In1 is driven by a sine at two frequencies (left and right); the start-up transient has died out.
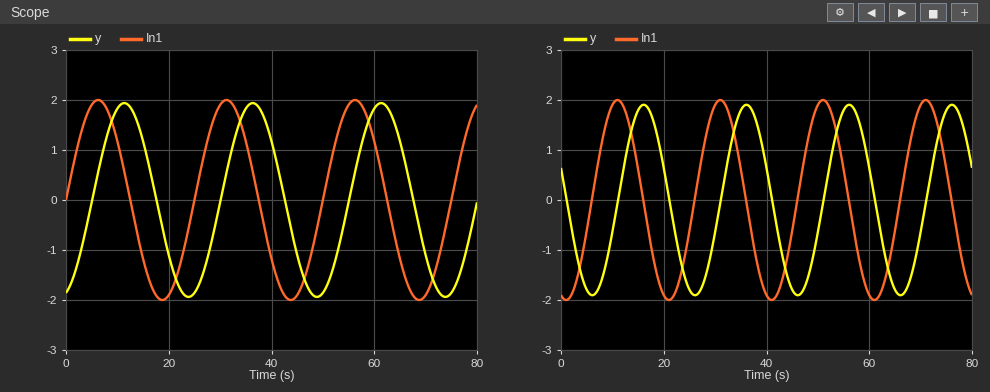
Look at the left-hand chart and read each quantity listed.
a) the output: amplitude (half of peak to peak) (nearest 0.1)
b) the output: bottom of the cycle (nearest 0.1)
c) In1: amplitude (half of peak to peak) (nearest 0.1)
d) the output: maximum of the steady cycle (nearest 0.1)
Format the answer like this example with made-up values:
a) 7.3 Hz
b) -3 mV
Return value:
a) 1.9
b) -1.9
c) 2.0
d) 1.9
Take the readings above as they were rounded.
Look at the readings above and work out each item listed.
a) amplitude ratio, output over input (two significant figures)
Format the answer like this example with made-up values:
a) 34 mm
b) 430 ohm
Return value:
a) 0.95
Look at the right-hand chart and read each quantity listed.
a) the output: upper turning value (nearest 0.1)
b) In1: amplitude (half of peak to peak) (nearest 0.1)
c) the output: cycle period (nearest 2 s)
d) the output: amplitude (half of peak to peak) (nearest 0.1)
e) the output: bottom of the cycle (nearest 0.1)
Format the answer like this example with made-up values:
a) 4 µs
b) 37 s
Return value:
a) 1.9
b) 2.0
c) 20 s
d) 1.9
e) -1.9
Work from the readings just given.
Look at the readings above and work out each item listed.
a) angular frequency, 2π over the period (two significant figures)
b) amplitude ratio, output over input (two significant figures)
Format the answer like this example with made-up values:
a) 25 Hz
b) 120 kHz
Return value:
a) 0.31 rad/s
b) 0.95
